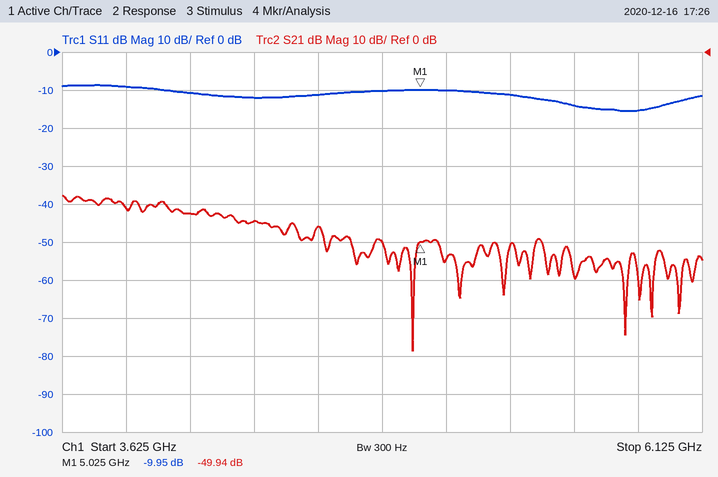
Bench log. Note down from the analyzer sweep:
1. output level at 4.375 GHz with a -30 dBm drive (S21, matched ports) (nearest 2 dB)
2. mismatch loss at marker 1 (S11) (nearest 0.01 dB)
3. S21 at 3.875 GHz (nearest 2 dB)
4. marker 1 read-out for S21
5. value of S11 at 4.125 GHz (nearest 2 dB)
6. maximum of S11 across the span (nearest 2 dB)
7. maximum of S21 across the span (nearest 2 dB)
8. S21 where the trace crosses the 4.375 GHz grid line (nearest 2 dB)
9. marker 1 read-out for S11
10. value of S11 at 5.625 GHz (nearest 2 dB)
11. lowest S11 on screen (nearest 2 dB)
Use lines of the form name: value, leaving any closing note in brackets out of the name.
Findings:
output level at 4.375 GHz with a -30 dBm drive (S21, matched ports): -74 dBm
mismatch loss at marker 1 (S11): 0.46 dB
S21 at 3.875 GHz: -42 dB
marker 1 read-out for S21: -49.94 dB
value of S11 at 4.125 GHz: -10 dB
maximum of S11 across the span: -8 dB
maximum of S21 across the span: -38 dB
S21 where the trace crosses the 4.375 GHz grid line: -44 dB
marker 1 read-out for S11: -9.95 dB
value of S11 at 5.625 GHz: -14 dB
lowest S11 on screen: -16 dB
